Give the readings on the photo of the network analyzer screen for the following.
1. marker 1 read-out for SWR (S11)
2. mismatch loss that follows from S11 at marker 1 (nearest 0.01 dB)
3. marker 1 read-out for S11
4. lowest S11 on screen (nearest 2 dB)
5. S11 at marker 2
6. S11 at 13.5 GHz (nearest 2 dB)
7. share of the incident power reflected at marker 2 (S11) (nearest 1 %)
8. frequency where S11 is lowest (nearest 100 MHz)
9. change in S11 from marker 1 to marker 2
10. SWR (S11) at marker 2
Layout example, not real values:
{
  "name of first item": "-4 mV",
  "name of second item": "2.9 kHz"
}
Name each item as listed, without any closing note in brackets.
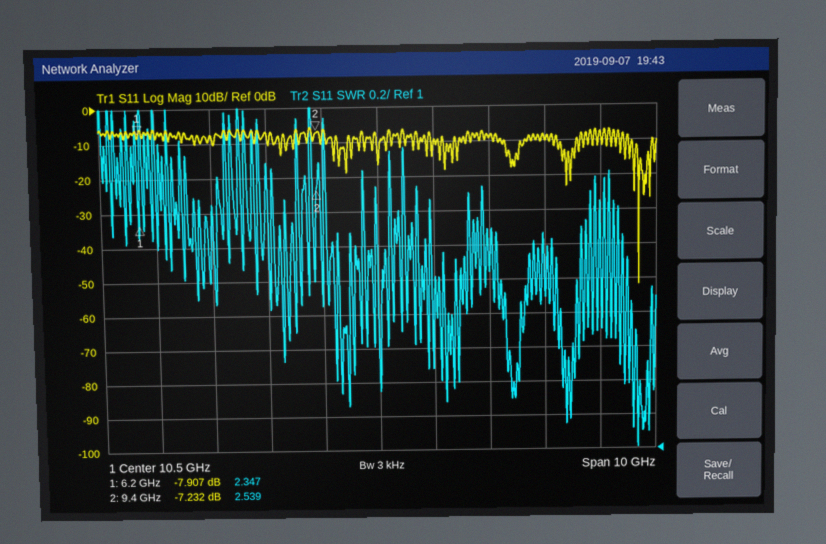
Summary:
{
  "marker 1 read-out for SWR": "2.347",
  "mismatch loss that follows from S11 at marker 1": "0.77 dB",
  "marker 1 read-out for S11": "-7.907 dB",
  "lowest S11 on screen": "-52 dB",
  "S11 at marker 2": "-7.232 dB",
  "S11 at 13.5 GHz": "-10 dB",
  "share of the incident power reflected at marker 2 (S11)": "19 %",
  "frequency where S11 is lowest": "15.2 GHz",
  "change in S11 from marker 1 to marker 2": "0.675 dB",
  "SWR (S11) at marker 2": "2.539"
}
